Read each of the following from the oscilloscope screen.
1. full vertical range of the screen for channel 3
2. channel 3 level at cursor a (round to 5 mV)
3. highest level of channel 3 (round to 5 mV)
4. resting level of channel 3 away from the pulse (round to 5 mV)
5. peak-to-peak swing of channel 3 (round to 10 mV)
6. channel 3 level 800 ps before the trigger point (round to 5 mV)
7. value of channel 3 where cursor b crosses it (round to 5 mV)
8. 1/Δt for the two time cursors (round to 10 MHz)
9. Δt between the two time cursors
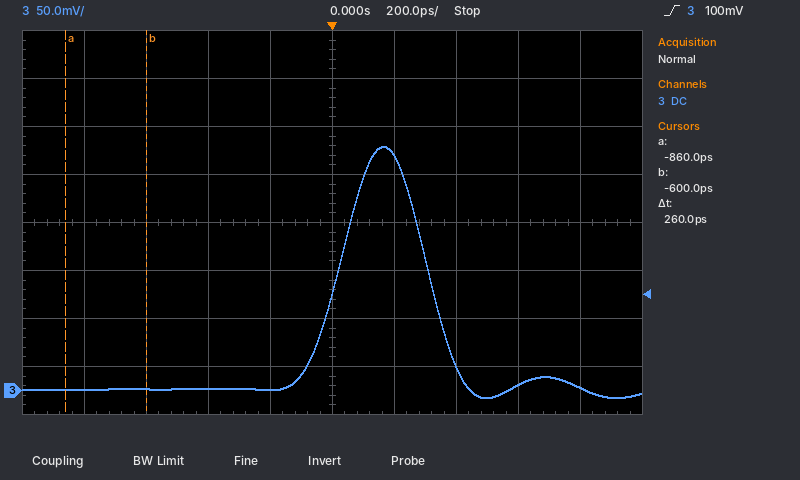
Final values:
400 mV
0 mV
255 mV
0 mV
260 mV
0 mV
0 mV
3.85 GHz
260 ps
